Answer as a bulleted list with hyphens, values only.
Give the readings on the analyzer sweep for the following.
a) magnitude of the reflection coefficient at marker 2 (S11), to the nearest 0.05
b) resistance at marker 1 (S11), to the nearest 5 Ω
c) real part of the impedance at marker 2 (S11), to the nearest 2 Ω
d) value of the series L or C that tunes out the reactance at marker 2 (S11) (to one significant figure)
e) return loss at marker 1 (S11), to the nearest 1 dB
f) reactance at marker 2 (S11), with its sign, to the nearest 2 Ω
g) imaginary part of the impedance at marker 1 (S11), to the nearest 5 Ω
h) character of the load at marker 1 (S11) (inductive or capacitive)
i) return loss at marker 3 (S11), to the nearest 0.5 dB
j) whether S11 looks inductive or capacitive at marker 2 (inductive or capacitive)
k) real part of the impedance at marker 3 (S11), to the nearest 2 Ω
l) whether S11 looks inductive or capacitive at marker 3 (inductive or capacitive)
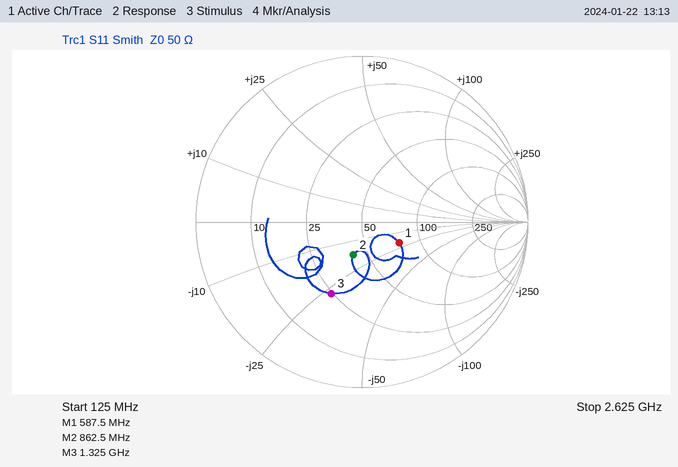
- 0.20
- 75 Ω
- 42 Ω
- 3 nH
- 12 dB
- -18 Ω
- -20 Ω
- capacitive
- 6.5 dB
- capacitive
- 24 Ω
- capacitive
